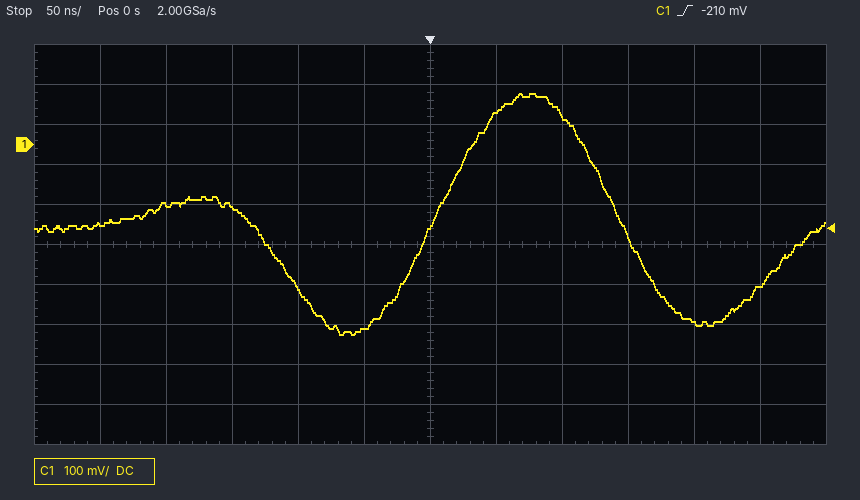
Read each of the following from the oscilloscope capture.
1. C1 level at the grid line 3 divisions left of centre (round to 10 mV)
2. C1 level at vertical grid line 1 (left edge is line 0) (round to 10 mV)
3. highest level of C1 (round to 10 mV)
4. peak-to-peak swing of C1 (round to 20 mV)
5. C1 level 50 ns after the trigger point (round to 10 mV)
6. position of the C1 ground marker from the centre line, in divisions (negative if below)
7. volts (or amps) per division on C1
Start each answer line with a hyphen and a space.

- -150 mV
- -200 mV
- 130 mV
- 600 mV
- 80 mV
- +2.5 div
- 100 mV
